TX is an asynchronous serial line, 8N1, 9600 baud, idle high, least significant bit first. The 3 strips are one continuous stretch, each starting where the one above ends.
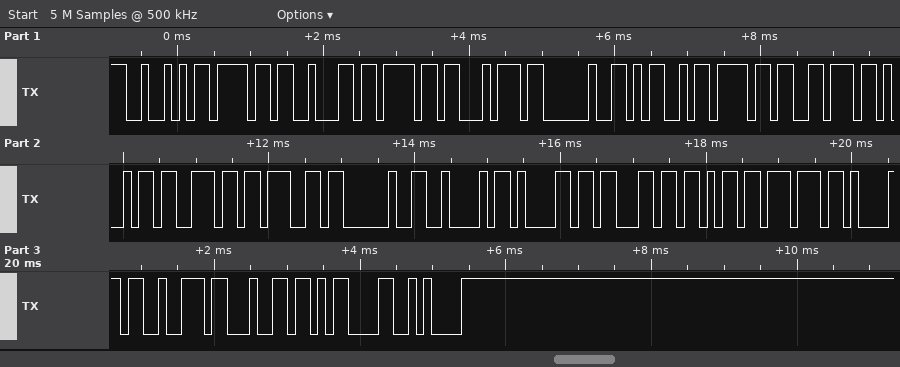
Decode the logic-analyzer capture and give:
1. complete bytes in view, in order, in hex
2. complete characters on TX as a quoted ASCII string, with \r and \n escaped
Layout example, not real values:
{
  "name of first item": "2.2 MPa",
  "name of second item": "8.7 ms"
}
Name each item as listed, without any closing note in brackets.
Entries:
{
  "complete bytes in view, in order, in hex": "52 6F 62 6F 74 20 4D 6F 76 69 6E 67 20 42 61 63 6B 77 61 72 64 0D 0A",
  "complete characters on TX as a quoted ASCII string, with \\r and \\n escaped": "\"Robot Moving Backward\\r\\n\""
}
